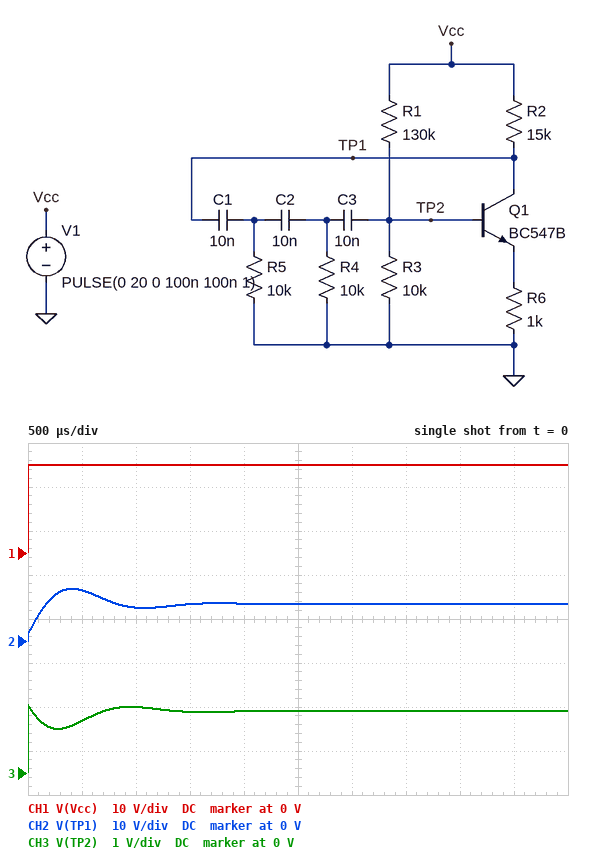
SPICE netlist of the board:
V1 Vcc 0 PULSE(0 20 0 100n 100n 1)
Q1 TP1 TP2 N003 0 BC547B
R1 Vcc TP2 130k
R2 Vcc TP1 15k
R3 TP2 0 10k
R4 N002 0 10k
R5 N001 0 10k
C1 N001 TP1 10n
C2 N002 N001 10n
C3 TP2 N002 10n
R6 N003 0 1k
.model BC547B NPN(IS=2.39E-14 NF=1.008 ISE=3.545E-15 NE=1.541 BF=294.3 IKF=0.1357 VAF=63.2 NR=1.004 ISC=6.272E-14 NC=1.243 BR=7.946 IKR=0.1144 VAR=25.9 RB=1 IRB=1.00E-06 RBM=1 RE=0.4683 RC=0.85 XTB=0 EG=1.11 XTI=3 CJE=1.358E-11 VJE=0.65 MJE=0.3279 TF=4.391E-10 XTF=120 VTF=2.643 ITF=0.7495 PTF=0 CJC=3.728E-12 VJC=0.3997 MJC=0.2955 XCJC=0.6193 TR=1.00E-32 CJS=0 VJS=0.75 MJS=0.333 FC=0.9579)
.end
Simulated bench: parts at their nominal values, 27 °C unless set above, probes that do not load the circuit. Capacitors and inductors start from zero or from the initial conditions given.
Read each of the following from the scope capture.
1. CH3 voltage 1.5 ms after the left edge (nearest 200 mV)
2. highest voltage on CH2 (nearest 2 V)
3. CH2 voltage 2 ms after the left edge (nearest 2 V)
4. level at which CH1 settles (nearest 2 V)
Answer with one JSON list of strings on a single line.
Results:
["1.4 V", "12 V", "8 V", "20 V"]
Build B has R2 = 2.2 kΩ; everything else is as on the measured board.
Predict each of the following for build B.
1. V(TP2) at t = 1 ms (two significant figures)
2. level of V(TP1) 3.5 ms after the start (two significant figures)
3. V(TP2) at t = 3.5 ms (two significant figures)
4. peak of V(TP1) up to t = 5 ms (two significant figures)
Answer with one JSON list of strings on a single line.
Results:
["1.4 V", "18 V", "1.4 V", "20 V"]
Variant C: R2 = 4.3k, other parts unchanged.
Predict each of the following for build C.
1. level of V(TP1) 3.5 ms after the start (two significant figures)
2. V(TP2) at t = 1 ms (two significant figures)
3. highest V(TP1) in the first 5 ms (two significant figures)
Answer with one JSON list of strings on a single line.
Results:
["17 V", "1.4 V", "19 V"]
